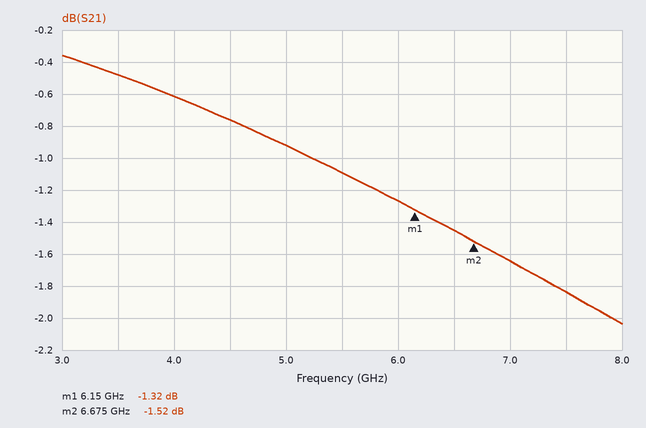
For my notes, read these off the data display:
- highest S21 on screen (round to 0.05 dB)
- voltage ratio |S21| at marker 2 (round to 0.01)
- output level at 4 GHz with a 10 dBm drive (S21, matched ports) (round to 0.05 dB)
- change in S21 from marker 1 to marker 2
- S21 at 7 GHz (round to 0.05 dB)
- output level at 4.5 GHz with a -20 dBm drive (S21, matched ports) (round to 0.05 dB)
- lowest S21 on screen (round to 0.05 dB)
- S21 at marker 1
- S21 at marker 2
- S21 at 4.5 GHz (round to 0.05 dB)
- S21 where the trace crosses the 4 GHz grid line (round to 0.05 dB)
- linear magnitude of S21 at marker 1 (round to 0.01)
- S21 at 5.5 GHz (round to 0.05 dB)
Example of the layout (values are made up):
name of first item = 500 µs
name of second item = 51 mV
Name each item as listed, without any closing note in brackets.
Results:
highest S21 on screen = -0.35 dB
voltage ratio |S21| at marker 2 = 0.84
output level at 4 GHz with a 10 dBm drive (S21, matched ports) = 9.40 dBm
change in S21 from marker 1 to marker 2 = -0.20 dB
S21 at 7 GHz = -1.65 dB
output level at 4.5 GHz with a -20 dBm drive (S21, matched ports) = -20.75 dBm
lowest S21 on screen = -2.05 dB
S21 at marker 1 = -1.32 dB
S21 at marker 2 = -1.52 dB
S21 at 4.5 GHz = -0.75 dB
S21 where the trace crosses the 4 GHz grid line = -0.60 dB
linear magnitude of S21 at marker 1 = 0.86
S21 at 5.5 GHz = -1.10 dB
